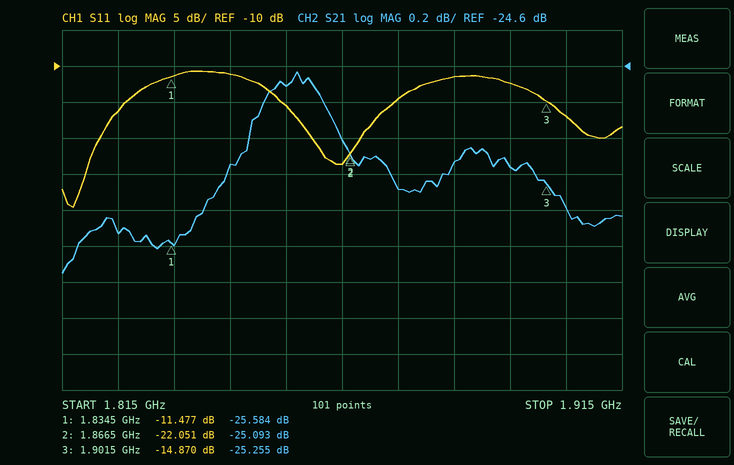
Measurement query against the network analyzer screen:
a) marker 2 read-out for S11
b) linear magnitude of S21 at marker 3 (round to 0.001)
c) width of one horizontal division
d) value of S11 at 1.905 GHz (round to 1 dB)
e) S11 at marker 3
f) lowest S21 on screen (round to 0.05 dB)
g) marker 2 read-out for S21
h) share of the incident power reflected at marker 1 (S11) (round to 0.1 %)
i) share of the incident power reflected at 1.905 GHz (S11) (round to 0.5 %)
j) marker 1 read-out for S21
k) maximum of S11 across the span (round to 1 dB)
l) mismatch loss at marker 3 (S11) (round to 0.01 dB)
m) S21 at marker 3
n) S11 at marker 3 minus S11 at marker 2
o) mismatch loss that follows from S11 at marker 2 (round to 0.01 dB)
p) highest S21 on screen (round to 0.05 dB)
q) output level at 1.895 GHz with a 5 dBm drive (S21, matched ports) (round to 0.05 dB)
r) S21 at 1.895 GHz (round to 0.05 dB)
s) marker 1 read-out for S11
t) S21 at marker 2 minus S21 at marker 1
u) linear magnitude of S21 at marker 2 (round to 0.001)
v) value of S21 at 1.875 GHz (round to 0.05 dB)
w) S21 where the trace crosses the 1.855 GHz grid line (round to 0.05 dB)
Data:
-22.051 dB
0.055
10 MHz
-17 dB
-14.870 dB
-25.75 dB
-25.093 dB
7.1 %
2.0 %
-25.584 dB
-11 dB
0.14 dB
-25.255 dB
7.181 dB
0.03 dB
-24.65 dB
-20.15 dBm
-25.15 dB
-11.477 dB
0.491 dB
0.056
-25.30 dB
-24.70 dB
